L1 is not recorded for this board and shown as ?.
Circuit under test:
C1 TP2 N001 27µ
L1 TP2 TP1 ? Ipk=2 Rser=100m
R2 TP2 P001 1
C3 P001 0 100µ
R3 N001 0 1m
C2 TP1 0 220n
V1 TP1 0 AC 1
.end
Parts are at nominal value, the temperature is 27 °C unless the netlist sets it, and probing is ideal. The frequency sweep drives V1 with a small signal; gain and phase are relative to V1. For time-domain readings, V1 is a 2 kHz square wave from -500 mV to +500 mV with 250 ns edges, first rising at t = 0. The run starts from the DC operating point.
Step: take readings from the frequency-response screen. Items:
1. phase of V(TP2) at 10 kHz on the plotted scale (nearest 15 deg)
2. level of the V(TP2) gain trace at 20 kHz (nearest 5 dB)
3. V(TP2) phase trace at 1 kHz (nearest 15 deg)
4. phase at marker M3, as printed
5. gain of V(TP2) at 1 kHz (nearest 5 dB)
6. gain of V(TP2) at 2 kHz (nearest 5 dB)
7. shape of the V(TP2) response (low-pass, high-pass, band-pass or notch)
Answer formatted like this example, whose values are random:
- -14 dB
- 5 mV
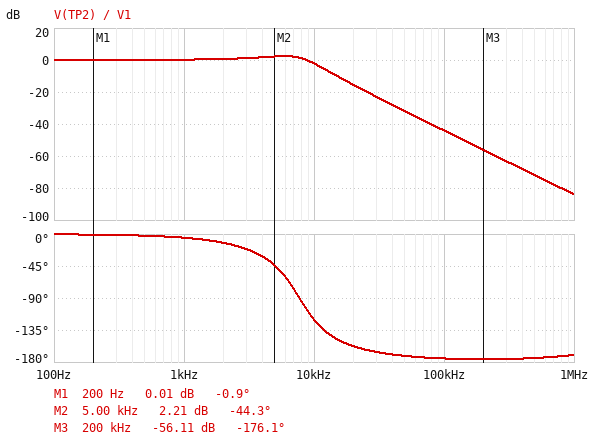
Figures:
- -120 deg
- -15 dB
- 0 deg
- -176.1 deg
- 0 dB
- 0 dB
- low-pass
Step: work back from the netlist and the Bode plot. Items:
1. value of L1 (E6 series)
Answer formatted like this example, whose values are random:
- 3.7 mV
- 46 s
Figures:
- 15 µH
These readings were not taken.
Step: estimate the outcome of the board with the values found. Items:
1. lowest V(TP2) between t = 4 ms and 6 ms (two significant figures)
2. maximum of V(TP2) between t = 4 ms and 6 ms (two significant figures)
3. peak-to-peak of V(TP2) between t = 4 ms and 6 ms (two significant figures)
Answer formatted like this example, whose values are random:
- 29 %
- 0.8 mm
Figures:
- -760 mV
- 760 mV
- 1.5 V
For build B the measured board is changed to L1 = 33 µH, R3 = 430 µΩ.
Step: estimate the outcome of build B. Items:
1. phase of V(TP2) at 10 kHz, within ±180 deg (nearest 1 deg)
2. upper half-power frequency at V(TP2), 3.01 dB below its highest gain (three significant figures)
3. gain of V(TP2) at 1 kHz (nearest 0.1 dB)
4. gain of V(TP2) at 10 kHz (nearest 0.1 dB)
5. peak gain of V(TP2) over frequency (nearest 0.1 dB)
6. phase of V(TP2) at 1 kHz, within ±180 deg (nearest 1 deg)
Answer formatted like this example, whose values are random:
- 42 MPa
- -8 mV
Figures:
- -141 deg
- 5.08 kHz
- 0.8 dB
- -10.9 dB
- 2.3 dB
- -8 deg
